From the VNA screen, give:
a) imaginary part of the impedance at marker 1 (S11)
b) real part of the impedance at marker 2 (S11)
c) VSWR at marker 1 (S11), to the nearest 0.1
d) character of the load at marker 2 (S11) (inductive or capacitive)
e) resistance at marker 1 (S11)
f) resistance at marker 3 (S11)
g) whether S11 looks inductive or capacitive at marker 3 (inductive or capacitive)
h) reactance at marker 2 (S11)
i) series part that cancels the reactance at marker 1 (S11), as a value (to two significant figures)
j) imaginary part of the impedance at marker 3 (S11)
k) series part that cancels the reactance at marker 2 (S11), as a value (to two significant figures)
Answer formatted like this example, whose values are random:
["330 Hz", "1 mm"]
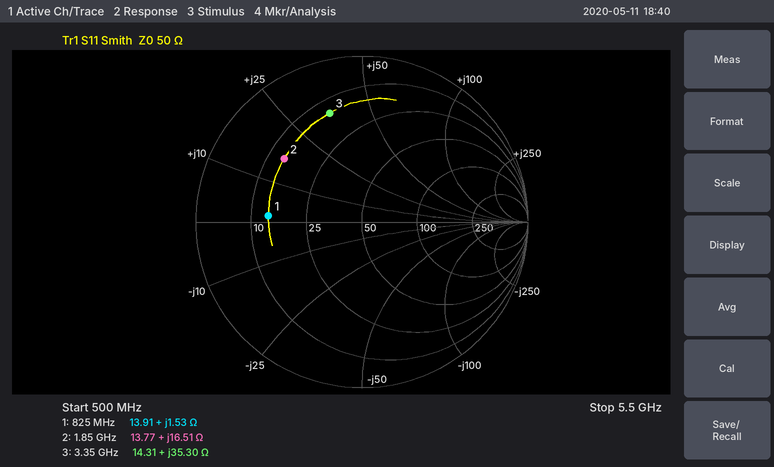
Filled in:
["+1.53 Ω", "13.77 Ω", "3.6", "inductive", "13.91 Ω", "14.31 Ω", "inductive", "+16.51 Ω", "130 pF", "+35.30 Ω", "5.2 pF"]
